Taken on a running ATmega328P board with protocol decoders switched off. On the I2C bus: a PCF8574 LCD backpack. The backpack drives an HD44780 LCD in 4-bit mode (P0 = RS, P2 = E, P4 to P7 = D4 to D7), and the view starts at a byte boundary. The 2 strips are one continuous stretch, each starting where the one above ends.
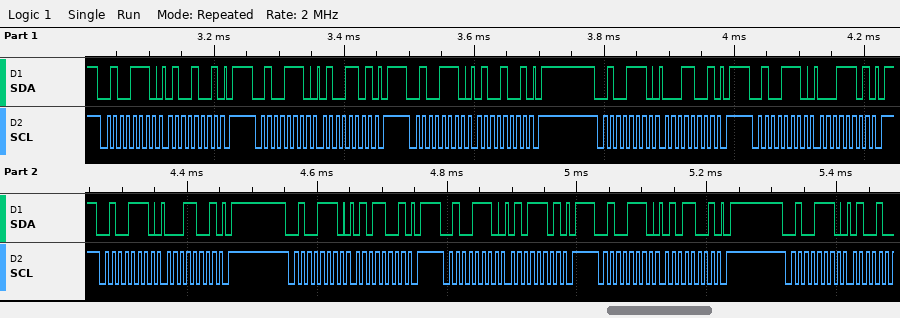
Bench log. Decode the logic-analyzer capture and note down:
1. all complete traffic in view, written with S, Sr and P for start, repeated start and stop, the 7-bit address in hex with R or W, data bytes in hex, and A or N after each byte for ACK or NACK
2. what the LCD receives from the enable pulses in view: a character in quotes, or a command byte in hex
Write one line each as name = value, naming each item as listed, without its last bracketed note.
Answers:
all complete traffic in view, written with S, Sr and P for start, repeated start and stop, the 7-bit address in hex with R or W, data bytes in hex, and A or N after each byte for ACK or NACK = S 27W A 49 A P S 27W A 4D A P S 27W A 49 A P S 27W A 19 A P S 27W A 1D A P S 27W A 19 A P S 27W A 59 A P S 27W A 5D A P S 27W A 59 A P S 27W A
what the LCD receives from the enable pulses in view: a character in quotes, or a command byte in hex = 'A'
